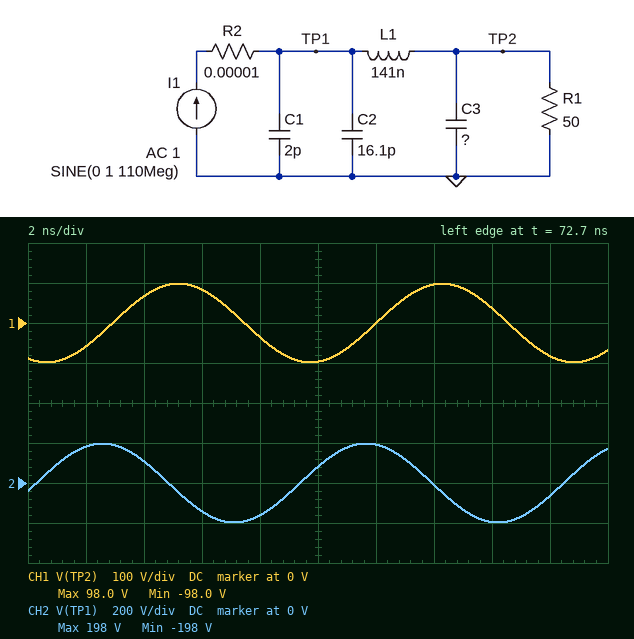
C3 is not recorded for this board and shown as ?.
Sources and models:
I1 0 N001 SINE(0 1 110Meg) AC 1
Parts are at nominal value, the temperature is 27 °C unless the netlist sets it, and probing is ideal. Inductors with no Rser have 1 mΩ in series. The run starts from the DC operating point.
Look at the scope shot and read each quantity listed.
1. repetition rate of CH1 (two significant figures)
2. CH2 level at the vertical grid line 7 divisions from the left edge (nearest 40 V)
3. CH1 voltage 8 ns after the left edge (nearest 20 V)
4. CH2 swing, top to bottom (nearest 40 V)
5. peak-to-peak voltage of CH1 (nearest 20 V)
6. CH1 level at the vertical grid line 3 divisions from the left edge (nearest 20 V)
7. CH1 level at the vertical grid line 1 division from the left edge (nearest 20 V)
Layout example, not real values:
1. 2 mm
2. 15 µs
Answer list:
1. 110 MHz
2. 0 V
3. -40 V
4. 400 V
5. 200 V
6. 80 V
7. -60 V
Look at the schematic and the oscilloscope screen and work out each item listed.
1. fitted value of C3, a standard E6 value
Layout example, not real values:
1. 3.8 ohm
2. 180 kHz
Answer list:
1. 22 pF
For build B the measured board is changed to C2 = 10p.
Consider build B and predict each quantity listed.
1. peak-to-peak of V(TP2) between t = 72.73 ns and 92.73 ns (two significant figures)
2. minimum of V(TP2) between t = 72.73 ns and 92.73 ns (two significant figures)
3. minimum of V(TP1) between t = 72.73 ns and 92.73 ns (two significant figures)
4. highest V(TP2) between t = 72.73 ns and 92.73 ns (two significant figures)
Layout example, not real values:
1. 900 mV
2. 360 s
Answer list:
1. 170 V
2. -84 V
3. -170 V
4. 84 V
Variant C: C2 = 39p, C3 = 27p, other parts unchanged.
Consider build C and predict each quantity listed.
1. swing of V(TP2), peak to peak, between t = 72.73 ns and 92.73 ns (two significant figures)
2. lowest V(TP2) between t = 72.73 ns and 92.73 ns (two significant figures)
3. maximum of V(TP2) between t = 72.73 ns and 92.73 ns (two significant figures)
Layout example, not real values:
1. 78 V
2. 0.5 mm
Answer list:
1. 56 V
2. -28 V
3. 28 V
